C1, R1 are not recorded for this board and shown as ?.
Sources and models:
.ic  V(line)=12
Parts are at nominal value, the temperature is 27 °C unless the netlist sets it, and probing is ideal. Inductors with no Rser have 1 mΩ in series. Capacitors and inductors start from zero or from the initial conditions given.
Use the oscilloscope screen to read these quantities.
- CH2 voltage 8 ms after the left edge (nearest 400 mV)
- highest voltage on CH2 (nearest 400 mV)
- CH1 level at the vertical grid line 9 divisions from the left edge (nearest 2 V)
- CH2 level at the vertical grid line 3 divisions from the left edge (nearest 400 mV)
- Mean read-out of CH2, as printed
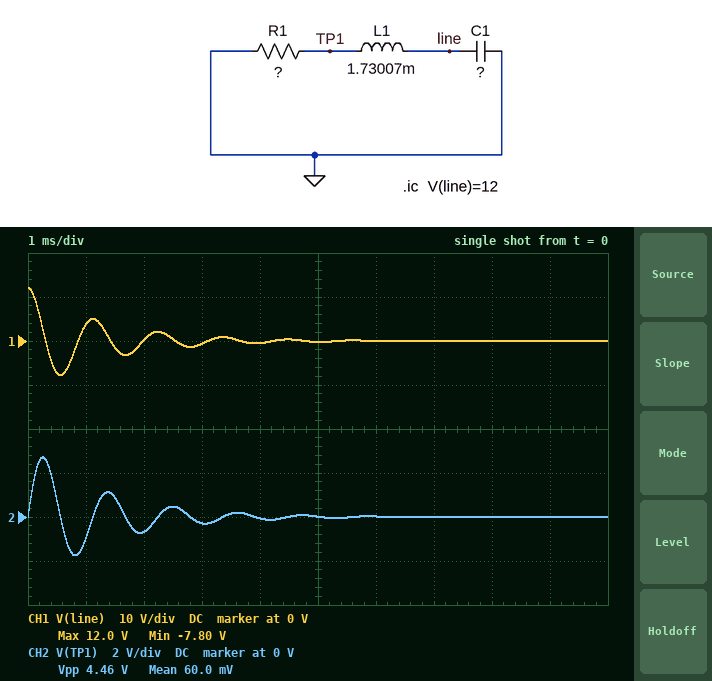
0 V
2.8 V
0 V
-400 mV
60.0 mV
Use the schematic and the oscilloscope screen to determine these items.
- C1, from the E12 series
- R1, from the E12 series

18 µF
2.7 Ω
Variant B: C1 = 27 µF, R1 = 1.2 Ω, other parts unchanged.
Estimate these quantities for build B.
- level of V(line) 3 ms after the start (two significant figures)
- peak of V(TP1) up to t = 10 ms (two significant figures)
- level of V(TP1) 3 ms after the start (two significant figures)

1.5 V
1.6 V
610 mV
